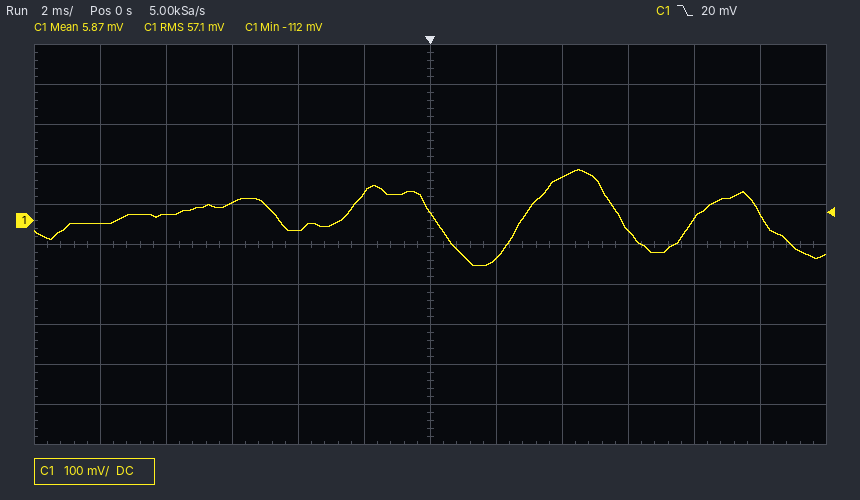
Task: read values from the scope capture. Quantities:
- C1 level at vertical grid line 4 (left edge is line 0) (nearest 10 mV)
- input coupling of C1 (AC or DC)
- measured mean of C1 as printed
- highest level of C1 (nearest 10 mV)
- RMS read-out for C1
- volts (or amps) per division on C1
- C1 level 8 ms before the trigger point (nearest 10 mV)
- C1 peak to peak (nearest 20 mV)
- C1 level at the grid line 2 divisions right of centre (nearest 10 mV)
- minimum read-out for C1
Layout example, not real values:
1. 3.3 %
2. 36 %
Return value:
1. -20 mV
2. DC
3. 5.87 mV
4. 130 mV
5. 57.1 mV
6. 100 mV
7. 20 mV
8. 240 mV
9. 110 mV
10. -112 mV
